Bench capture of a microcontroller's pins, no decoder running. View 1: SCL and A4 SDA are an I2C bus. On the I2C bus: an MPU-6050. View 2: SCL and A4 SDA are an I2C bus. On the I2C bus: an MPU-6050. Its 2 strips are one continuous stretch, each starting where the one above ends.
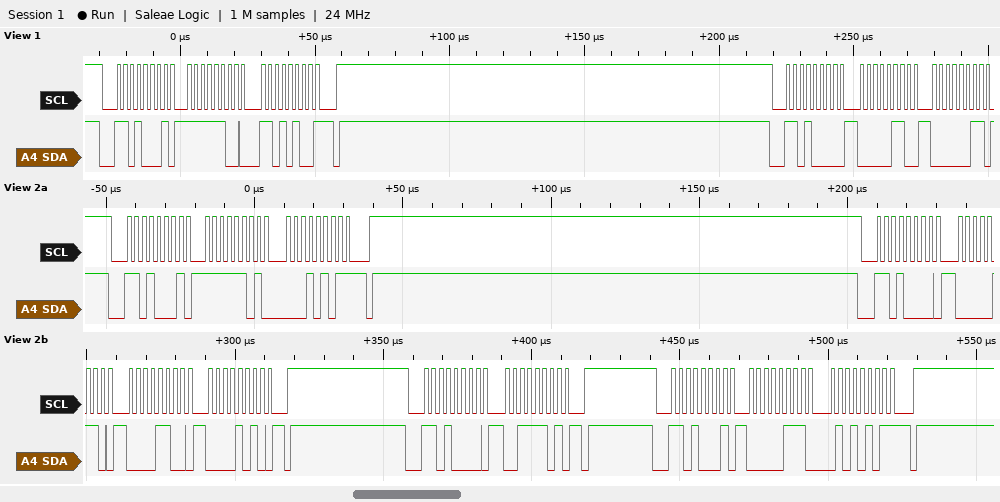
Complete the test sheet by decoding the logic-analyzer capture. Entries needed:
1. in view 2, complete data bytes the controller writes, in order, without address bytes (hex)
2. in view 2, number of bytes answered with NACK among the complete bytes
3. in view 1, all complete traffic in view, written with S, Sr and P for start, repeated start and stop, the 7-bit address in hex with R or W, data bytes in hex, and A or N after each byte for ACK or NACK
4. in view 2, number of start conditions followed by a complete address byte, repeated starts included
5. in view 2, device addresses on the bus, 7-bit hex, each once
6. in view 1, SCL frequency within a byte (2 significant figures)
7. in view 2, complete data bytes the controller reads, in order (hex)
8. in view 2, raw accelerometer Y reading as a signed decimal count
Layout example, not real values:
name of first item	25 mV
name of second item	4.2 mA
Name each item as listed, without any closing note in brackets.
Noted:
in view 2, complete data bytes the controller writes, in order, without address bytes	06 0C 0A 3D
in view 2, number of bytes answered with NACK among the complete bytes	2
in view 1, all complete traffic in view, written with S, Sr and P for start, repeated start and stop, the 7-bit address in hex with R or W, data bytes in hex, and A or N after each byte for ACK or NACK	S 68R A FC A D4 N P S 68W A 06 A 03 A
in view 2, number of start conditions followed by a complete address byte, repeated starts included	4
in view 2, device addresses on the bus, 7-bit hex, each once	0x68
in view 1, SCL frequency within a byte	400 kHz
in view 2, complete data bytes the controller reads, in order	FD 15 07 55
in view 2, raw accelerometer Y reading as a signed decimal count	1877
